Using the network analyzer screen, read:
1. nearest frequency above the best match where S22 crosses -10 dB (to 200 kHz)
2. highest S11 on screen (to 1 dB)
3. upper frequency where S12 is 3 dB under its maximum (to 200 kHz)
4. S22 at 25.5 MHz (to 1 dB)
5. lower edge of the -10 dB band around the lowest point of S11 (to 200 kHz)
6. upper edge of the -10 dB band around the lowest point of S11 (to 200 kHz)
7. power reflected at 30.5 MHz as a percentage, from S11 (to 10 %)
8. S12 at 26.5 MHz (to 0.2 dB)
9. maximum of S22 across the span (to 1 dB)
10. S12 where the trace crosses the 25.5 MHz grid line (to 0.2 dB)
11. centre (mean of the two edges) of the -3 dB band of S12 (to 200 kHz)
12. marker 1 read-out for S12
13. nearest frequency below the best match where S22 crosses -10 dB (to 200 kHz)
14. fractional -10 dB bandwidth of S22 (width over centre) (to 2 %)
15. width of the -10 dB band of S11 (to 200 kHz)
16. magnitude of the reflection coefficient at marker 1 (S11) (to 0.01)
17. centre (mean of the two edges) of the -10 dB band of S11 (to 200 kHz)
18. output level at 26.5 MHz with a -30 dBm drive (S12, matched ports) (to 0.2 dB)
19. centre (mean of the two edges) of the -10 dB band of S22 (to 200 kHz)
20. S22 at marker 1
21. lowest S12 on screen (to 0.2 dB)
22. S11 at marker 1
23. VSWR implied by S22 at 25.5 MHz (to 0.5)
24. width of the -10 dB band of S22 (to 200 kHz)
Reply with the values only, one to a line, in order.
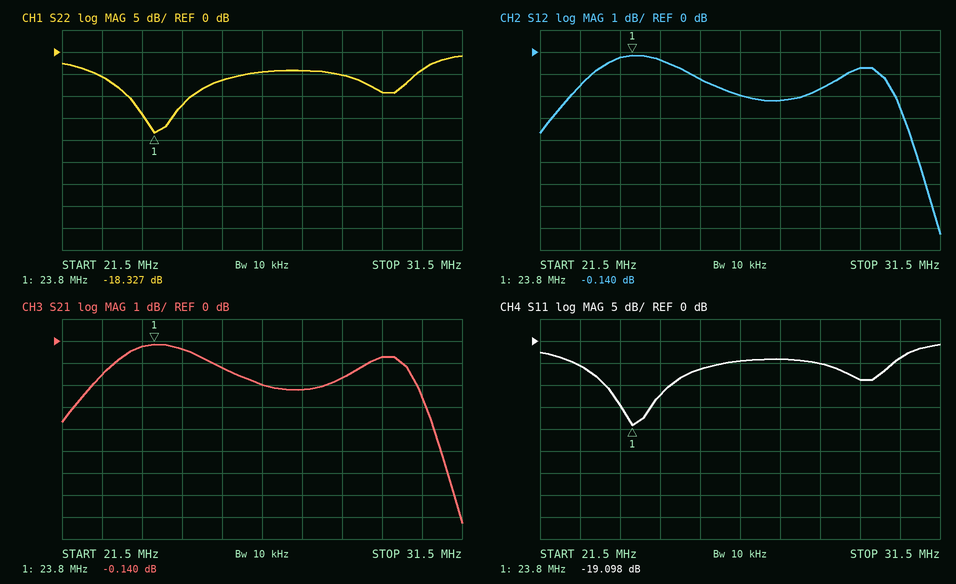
24.8 MHz
-1 dB
30.6 MHz
-6 dB
23.2 MHz
24.8 MHz
40 %
-2.0 dB
-1 dB
-1.2 dB
26.2 MHz
-0.140 dB
23.2 MHz
6 %
1.6 MHz
0.11
24.0 MHz
-32.0 dBm
24.0 MHz
-18.327 dB
-8.2 dB
-19.098 dB
3.0
1.6 MHz
